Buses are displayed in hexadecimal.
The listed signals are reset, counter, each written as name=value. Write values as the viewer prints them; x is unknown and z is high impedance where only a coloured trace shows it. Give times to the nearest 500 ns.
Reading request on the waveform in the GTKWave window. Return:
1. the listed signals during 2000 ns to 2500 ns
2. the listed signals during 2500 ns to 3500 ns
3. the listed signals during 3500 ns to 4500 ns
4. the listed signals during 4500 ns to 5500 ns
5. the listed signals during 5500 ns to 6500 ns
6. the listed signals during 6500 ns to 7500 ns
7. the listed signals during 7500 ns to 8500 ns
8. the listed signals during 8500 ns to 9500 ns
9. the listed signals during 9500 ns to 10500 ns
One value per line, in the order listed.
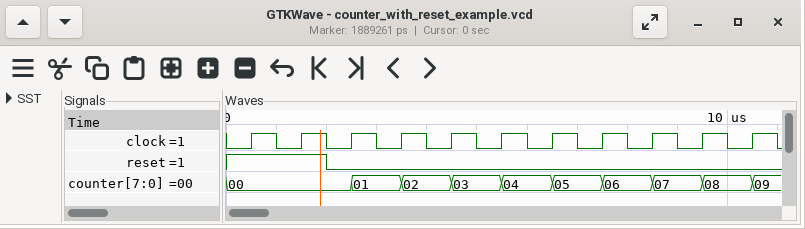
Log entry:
reset=0, counter=00
reset=0, counter=01
reset=0, counter=02
reset=0, counter=03
reset=0, counter=04
reset=0, counter=05
reset=0, counter=06
reset=0, counter=07
reset=0, counter=08
